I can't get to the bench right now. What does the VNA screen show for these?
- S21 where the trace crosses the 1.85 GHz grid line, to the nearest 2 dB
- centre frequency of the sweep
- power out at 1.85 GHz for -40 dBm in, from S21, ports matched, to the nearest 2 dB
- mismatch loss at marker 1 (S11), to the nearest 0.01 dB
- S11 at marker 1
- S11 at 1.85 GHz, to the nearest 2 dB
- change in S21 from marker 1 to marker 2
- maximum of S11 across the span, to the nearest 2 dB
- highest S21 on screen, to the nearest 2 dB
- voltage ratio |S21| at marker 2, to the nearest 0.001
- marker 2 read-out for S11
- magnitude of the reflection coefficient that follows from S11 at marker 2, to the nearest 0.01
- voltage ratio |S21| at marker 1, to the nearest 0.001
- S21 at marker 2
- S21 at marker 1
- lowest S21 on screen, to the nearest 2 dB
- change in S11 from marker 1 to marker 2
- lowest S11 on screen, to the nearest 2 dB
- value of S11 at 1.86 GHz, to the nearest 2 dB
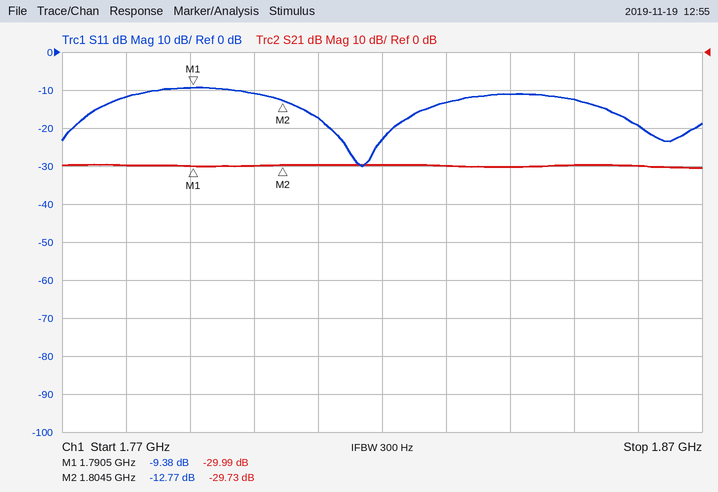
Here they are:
-30 dB
1.82 GHz
-70 dBm
0.53 dB
-9.38 dB
-12 dB
0.26 dB
-10 dB
-30 dB
0.033
-12.77 dB
0.23
0.032
-29.73 dB
-29.99 dB
-30 dB
-3.39 dB
-30 dB
-20 dB
